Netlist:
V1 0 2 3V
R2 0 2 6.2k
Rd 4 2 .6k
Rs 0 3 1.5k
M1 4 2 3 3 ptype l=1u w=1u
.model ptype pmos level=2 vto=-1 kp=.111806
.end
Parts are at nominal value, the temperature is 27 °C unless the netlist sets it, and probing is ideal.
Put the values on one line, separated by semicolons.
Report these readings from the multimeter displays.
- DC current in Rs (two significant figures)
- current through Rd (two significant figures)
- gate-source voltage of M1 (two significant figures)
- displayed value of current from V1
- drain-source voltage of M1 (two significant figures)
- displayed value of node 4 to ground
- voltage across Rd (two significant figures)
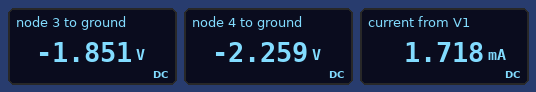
1.2 mA; 1.2 mA; -1.1 V; 1.718 mA; -410 mV; -2.259 V; 740 mV
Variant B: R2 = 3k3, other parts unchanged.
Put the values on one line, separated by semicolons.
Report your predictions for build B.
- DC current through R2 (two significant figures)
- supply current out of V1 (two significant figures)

910 µA; 2.1 mA
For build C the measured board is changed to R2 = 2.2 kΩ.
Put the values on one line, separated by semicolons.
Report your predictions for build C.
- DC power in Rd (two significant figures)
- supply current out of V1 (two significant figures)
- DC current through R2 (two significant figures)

910 µW; 2.6 mA; 1.4 mA
